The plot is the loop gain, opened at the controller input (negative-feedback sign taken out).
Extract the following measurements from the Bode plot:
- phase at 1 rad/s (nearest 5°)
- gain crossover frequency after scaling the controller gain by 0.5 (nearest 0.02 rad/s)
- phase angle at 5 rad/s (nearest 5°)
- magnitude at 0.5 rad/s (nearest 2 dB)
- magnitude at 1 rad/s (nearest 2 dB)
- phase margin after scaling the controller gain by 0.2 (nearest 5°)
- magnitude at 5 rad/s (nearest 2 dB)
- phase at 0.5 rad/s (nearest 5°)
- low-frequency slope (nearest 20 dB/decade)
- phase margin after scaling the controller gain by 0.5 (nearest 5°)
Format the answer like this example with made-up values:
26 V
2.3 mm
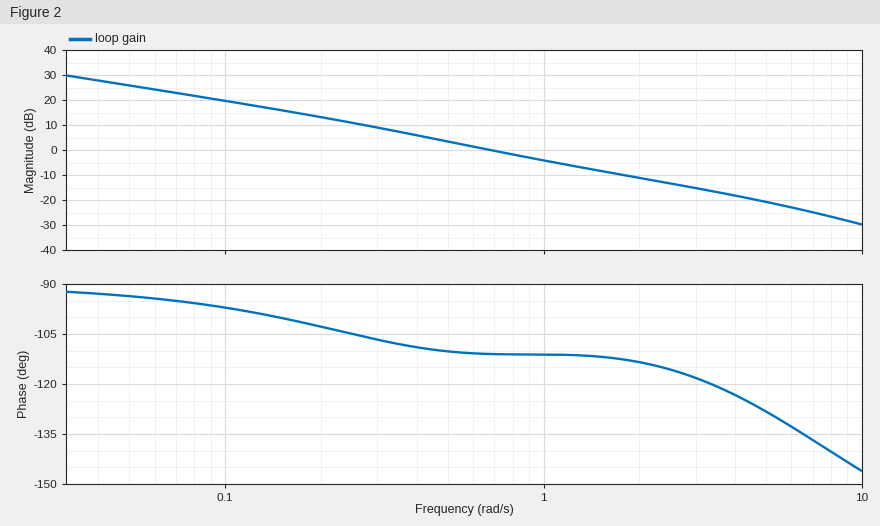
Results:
-110°
0.40 rad/s
-130°
4 dB
-4 dB
80°
-20 dB
-110°
-20 dB/decade
70°
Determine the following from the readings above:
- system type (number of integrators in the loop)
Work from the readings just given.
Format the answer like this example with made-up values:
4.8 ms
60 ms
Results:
1
